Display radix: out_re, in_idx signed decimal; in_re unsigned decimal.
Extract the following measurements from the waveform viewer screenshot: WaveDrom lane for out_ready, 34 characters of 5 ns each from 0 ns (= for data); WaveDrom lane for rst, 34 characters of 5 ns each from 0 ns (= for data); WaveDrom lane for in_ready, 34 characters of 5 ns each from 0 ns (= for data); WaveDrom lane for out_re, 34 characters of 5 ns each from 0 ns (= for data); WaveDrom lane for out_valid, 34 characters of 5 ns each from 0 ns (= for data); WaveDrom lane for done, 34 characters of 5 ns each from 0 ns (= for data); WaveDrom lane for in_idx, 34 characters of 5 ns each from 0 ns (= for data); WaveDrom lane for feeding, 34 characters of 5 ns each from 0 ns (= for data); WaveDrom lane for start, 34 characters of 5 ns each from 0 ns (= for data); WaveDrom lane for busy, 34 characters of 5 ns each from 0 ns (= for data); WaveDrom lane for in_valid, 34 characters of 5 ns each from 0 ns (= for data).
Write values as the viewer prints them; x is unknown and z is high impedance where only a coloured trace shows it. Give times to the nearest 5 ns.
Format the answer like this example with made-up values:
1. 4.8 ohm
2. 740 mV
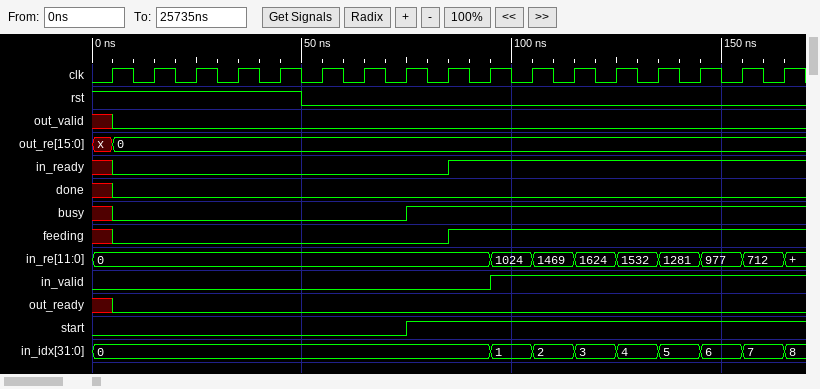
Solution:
1. {name: 'out_ready', wave: 'x0................................'}
2. {name: 'rst', wave: '1.........0.......................'}
3. {name: 'in_ready', wave: 'x0...............1................'}
4. {name: 'out_re', wave: 'x=................................', data: '0'}
5. {name: 'out_valid', wave: 'x0................................'}
6. {name: 'done', wave: 'x0................................'}
7. {name: 'in_idx', wave: '=..................=.=.=.=.=.=.=.=', data: '0 1 2 3 4 5 6 7 8'}
8. {name: 'feeding', wave: 'x0...............1................'}
9. {name: 'start', wave: '0..............1..................'}
10. {name: 'busy', wave: 'x0.............1..................'}
11. {name: 'in_valid', wave: '0..................1..............'}
